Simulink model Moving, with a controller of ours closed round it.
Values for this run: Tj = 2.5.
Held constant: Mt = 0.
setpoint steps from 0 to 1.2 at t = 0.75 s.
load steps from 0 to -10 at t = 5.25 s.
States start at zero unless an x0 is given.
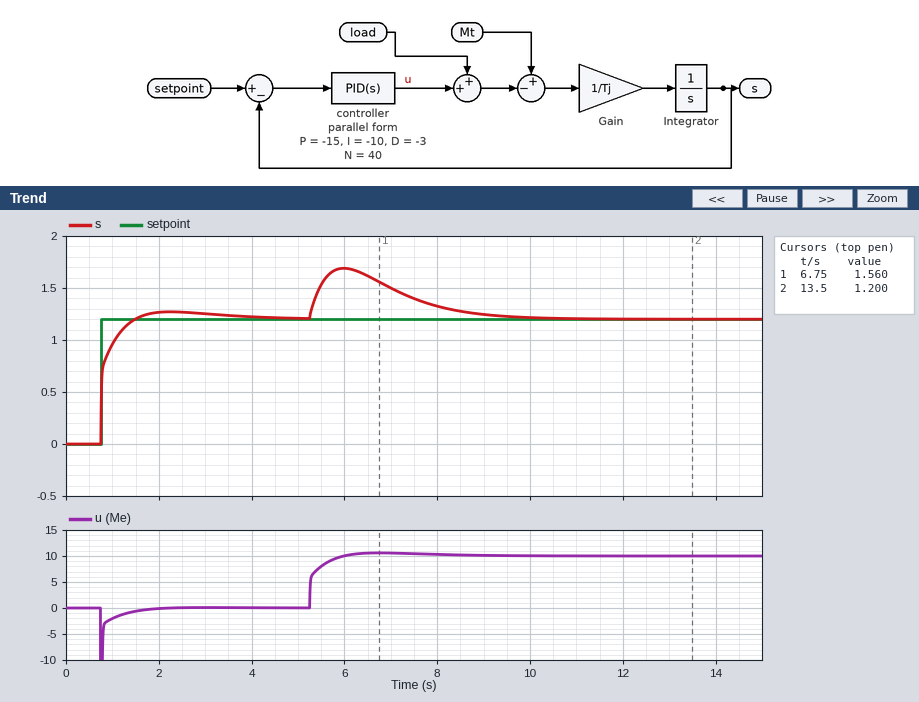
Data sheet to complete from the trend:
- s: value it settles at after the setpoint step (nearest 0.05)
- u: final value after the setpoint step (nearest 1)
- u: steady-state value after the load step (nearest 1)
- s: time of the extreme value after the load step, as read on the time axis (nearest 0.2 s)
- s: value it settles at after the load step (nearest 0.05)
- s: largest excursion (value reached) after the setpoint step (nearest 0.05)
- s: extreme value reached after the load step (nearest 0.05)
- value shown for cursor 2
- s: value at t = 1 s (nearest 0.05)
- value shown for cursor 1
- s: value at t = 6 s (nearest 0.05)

1.20
0
10
6.0 s
1.20
1.25
1.70
1.200
0.95
1.560
1.70
